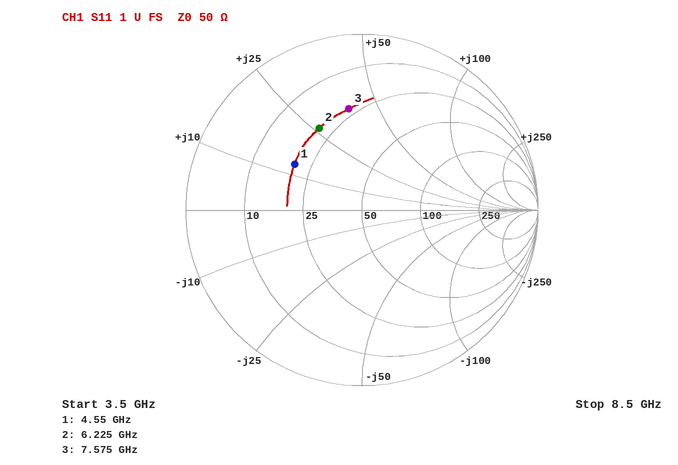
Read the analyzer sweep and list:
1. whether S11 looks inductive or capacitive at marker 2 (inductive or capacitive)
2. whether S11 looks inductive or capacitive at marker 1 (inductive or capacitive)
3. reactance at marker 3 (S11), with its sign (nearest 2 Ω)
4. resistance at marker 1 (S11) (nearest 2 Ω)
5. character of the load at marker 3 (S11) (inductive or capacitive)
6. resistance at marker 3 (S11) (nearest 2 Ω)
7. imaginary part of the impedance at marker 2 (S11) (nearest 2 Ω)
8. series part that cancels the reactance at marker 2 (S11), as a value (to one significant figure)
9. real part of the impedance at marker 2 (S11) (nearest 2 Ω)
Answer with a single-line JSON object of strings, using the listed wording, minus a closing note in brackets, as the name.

{"whether S11 looks inductive or capacitive at marker 2": "inductive", "whether S11 looks inductive or capacitive at marker 1": "inductive", "reactance at marker 3 (S11), with its sign": "+38 Ω", "resistance at marker 1 (S11)": "20 Ω", "character of the load at marker 3 (S11)": "inductive", "resistance at marker 3 (S11)": "22 Ω", "imaginary part of the impedance at marker 2 (S11)": "+26 Ω", "series part that cancels the reactance at marker 2 (S11), as a value": "1.0 pF", "real part of the impedance at marker 2 (S11)": "20 Ω"}
